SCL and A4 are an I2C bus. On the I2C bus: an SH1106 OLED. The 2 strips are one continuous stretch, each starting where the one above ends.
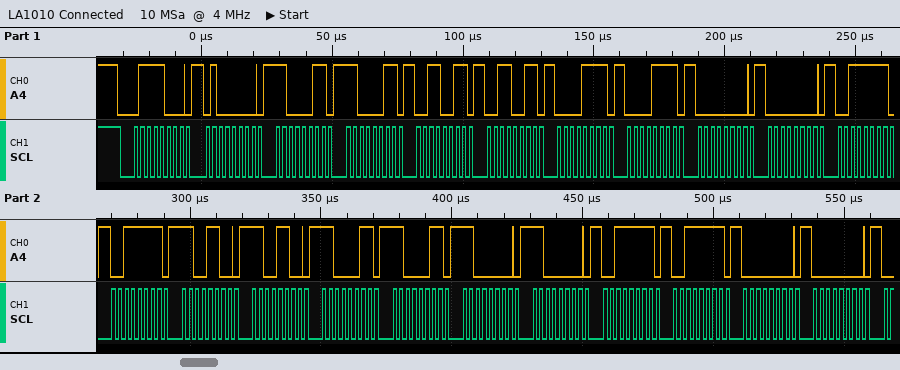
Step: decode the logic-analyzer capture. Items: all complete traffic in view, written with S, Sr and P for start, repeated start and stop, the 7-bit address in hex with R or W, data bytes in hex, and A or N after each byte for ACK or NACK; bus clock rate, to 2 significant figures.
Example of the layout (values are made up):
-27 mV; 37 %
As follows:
S 3CW A 40 A C3 A C3 A 33 A 33 A 0F A 0F A 00 A 00 A 3F A 3F A CC A CC A C3 A C3 A C0 A C0 A 3F A 3F A 00 A 00 A; 400 kHz
